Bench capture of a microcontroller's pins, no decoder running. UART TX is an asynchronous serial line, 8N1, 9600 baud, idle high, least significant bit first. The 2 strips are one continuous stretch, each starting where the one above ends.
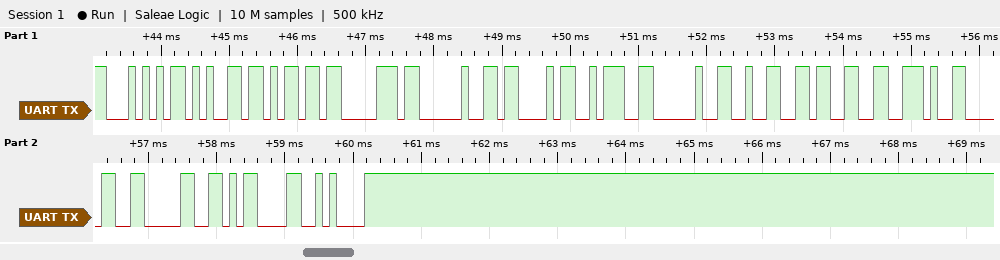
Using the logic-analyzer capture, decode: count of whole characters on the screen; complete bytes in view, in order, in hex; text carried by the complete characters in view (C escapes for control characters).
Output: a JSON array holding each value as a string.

["15", "54 65 6D 70 20 43 3A 20 32 33 2E 30 30 0D 0A", "\"Temp C: 23.00\\r\\n\""]
